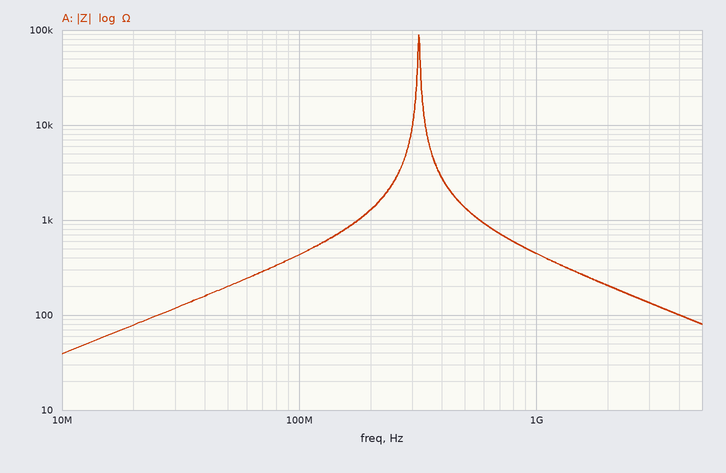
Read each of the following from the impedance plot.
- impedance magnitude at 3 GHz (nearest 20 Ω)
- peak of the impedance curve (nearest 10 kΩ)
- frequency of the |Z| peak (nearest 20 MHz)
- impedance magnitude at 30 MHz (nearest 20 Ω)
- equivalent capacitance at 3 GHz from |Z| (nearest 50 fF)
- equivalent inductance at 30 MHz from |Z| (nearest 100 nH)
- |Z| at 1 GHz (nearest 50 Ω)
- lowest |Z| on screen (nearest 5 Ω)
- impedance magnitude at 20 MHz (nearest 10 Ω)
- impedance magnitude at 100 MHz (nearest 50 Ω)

140 Ω
90 kΩ
320 MHz
120 Ω
400 fF
600 nH
450 Ω
40 Ω
80 Ω
450 Ω
